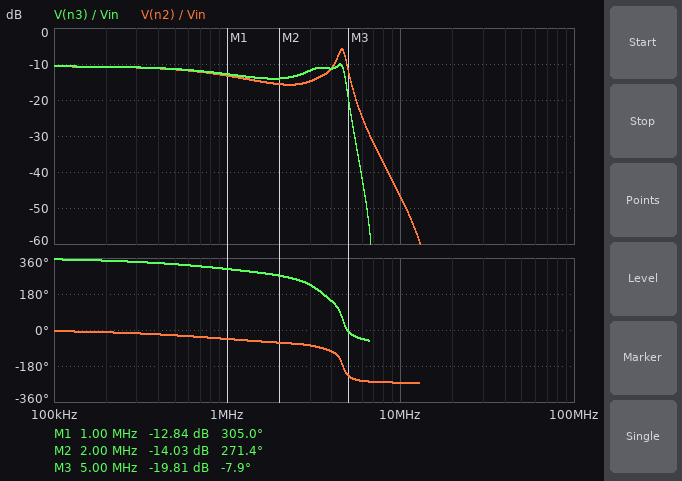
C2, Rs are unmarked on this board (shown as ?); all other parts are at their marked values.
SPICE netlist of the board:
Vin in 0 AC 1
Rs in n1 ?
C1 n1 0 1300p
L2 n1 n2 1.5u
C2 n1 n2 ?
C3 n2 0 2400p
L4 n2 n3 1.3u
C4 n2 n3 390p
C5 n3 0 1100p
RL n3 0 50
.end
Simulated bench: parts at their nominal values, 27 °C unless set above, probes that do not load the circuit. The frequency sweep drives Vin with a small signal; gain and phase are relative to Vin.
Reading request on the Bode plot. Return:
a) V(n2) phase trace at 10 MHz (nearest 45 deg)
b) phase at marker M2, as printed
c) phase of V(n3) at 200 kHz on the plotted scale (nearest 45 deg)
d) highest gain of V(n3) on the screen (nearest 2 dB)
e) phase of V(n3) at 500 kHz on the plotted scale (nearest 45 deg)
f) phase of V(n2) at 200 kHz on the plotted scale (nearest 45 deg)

-270 deg
271.4 deg
360 deg
-10 dB
315 deg
0 deg
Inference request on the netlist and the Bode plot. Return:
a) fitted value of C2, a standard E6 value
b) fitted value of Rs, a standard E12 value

68 pF
120 Ω
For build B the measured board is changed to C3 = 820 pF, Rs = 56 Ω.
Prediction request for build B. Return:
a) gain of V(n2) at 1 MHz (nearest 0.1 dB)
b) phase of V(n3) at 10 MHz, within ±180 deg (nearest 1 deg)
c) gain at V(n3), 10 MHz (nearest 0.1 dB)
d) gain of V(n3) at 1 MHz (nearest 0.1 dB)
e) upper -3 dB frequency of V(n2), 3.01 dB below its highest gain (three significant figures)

-7.3 dB
118 deg
-48.2 dB
-7.0 dB
6.00 MHz
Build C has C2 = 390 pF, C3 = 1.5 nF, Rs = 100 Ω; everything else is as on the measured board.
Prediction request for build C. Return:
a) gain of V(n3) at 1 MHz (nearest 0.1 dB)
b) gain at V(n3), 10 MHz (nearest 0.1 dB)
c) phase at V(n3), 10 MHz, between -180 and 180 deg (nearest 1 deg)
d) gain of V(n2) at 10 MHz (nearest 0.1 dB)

-10.8 dB
-54.8 dB
-70 deg
-38.1 dB
